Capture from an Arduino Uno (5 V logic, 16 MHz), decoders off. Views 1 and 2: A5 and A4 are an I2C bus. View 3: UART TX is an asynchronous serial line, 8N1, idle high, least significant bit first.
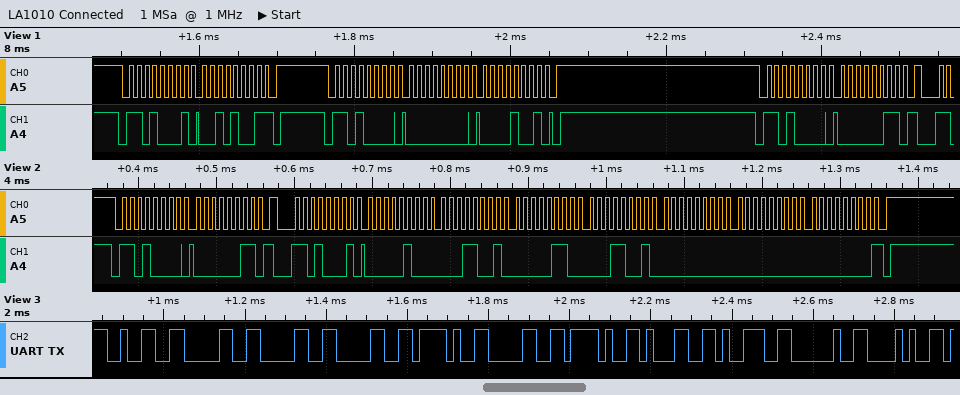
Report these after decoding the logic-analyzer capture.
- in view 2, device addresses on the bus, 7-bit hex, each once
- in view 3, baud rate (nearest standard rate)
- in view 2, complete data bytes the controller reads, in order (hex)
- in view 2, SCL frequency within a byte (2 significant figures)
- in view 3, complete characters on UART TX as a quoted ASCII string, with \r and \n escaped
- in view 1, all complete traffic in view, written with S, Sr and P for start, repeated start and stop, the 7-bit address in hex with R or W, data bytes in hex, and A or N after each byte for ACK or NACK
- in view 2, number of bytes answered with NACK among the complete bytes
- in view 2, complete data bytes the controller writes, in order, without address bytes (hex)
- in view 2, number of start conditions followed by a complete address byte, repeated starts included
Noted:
0x68
57600 baud
04 19 06 19 00 00 00
100 kHz
"2000/0/19 ("
S 68R A 29 N P S 68W A 00 A 09 A P S 68W A 03 A
1
03
2
